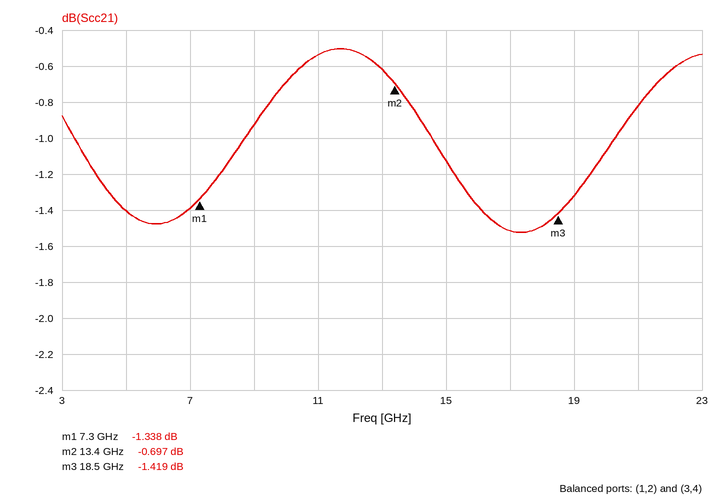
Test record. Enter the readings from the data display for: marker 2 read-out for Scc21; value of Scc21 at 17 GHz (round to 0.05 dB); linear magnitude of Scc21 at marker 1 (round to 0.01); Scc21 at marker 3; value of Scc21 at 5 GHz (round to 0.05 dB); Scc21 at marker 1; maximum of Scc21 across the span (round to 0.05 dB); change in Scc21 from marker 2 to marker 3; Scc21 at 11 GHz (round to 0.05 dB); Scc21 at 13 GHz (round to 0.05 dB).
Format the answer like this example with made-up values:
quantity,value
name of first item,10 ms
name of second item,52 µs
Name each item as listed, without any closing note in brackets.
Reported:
quantity,value
marker 2 read-out for Scc21,-0.697 dB
value of Scc21 at 17 GHz,-1.50 dB
linear magnitude of Scc21 at marker 1,0.86
Scc21 at marker 3,-1.419 dB
value of Scc21 at 5 GHz,-1.40 dB
Scc21 at marker 1,-1.338 dB
maximum of Scc21 across the span,-0.50 dB
change in Scc21 from marker 2 to marker 3,-0.722 dB
Scc21 at 11 GHz,-0.55 dB
Scc21 at 13 GHz,-0.60 dB
